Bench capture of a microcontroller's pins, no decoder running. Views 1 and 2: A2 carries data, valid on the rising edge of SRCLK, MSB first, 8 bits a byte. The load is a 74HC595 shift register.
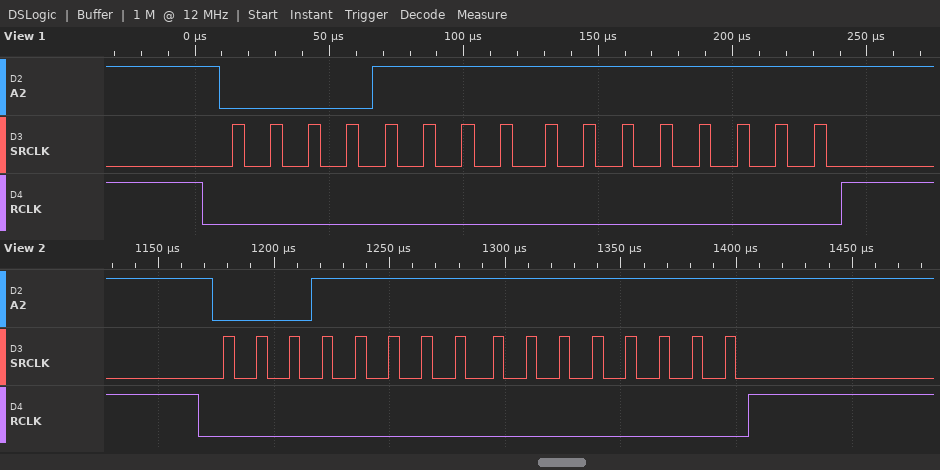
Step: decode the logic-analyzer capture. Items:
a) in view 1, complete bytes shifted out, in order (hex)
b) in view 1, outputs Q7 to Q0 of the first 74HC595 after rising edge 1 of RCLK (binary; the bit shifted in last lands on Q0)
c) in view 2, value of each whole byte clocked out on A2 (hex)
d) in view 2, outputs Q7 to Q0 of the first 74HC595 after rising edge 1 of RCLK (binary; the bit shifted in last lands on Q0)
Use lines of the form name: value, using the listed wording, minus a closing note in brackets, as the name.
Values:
in view 1, complete bytes shifted out, in order: 0x0F 0xFF
in view 1, outputs Q7 to Q0 of the first 74HC595 after rising edge 1 of RCLK: 11111111
in view 2, value of each whole byte clocked out on A2: 1F FF
in view 2, outputs Q7 to Q0 of the first 74HC595 after rising edge 1 of RCLK: 11111111
